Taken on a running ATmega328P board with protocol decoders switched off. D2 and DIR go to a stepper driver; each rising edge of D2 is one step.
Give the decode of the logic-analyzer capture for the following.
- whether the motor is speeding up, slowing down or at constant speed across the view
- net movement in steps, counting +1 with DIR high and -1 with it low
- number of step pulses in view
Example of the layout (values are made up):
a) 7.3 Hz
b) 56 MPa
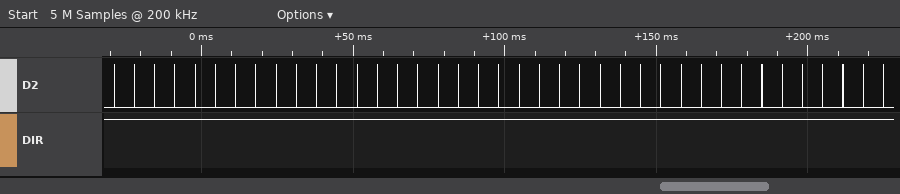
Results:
a) constant speed
b) +39
c) 39
